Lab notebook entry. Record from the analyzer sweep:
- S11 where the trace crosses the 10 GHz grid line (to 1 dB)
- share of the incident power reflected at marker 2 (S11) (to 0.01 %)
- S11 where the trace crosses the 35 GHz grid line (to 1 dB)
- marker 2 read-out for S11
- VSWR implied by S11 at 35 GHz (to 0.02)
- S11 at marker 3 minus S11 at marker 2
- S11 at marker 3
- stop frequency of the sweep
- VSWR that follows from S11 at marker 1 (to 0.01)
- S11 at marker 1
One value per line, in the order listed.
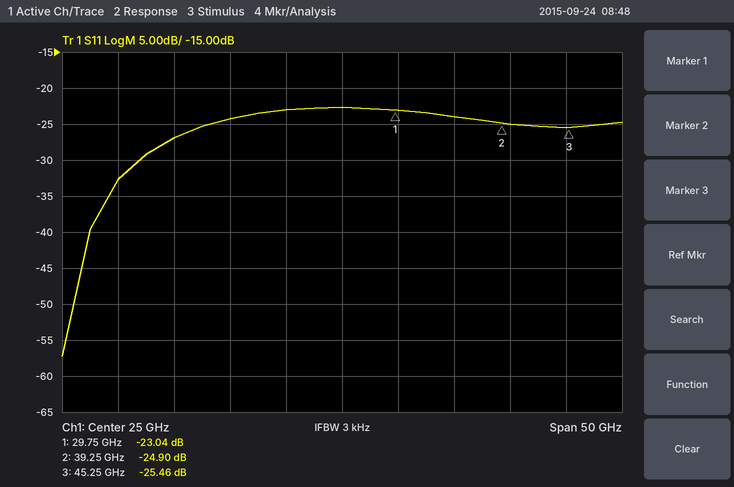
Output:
-27 dB
0.32 %
-24 dB
-24.90 dB
1.14
-0.56 dB
-25.46 dB
50 GHz
1.15
-23.04 dB
